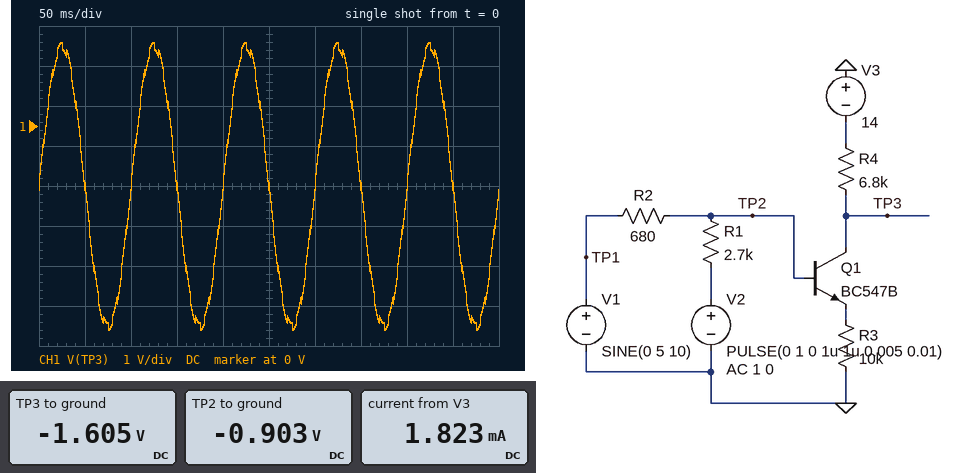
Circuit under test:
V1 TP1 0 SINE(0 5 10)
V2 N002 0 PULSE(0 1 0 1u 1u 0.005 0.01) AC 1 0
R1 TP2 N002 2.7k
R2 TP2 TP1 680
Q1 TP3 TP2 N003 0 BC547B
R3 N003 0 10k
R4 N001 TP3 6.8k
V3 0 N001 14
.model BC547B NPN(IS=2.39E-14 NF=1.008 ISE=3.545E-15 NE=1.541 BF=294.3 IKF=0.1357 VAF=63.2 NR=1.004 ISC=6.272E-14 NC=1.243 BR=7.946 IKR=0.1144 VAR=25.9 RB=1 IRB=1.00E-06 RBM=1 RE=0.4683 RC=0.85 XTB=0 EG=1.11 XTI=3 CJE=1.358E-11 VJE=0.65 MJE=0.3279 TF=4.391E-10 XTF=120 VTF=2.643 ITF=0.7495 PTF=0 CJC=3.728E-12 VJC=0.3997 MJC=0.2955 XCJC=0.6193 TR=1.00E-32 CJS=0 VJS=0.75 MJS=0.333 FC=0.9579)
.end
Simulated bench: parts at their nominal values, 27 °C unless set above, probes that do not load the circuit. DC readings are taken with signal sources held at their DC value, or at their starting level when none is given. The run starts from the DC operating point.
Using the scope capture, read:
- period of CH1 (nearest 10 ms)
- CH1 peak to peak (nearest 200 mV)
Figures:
100 ms
7.2 V
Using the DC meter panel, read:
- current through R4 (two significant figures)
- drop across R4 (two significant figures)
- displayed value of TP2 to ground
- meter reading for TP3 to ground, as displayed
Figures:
1.8 mA
12 V
-0.903 V
-1.605 V
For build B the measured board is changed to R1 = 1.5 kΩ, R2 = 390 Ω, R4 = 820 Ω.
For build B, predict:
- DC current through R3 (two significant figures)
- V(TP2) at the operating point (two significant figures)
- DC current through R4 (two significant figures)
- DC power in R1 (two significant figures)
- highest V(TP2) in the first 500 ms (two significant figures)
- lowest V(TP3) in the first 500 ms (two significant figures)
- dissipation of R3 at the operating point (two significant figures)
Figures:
430 µA
-3.5 V
12 mA
8.3 mW
-560 mV
-7.1 V
1.8 mW
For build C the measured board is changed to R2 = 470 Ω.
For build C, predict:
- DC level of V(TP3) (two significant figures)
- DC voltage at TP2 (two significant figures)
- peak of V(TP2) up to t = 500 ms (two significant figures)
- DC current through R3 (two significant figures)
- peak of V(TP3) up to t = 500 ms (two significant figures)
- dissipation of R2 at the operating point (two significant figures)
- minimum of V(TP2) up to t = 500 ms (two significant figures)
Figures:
-1.4 V
-690 mV
3.3 V
140 µA
2.6 V
1.0 mW
-4.6 V
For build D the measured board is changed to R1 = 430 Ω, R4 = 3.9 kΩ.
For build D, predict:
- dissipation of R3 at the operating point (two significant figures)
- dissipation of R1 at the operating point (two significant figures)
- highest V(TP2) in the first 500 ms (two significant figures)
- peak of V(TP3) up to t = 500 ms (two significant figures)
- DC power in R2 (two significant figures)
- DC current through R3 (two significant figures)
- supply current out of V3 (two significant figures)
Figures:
230 µW
1.5 mW
1.5 V
800 mV
950 µW
150 µA
3.2 mA
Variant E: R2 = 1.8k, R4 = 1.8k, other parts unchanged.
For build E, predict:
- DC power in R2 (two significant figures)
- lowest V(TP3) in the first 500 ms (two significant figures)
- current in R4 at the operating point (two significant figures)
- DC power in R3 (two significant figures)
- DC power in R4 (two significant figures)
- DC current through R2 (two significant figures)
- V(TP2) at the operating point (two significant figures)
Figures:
12 mW
-7.1 V
4.8 mA
2.9 mW
42 mW
2.6 mA
-4.6 V
